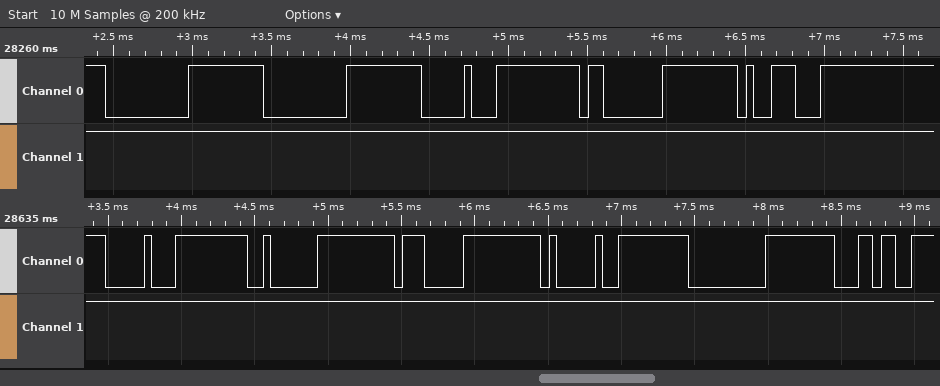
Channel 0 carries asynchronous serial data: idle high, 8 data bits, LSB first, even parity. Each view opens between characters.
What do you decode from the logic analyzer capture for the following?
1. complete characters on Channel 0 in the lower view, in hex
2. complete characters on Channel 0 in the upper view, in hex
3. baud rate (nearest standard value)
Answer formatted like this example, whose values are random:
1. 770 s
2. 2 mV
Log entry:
1. 10, 02, 07, 41, 00, 6C
2. 00, 00, 10, 03, 39
3. 19200 baud
